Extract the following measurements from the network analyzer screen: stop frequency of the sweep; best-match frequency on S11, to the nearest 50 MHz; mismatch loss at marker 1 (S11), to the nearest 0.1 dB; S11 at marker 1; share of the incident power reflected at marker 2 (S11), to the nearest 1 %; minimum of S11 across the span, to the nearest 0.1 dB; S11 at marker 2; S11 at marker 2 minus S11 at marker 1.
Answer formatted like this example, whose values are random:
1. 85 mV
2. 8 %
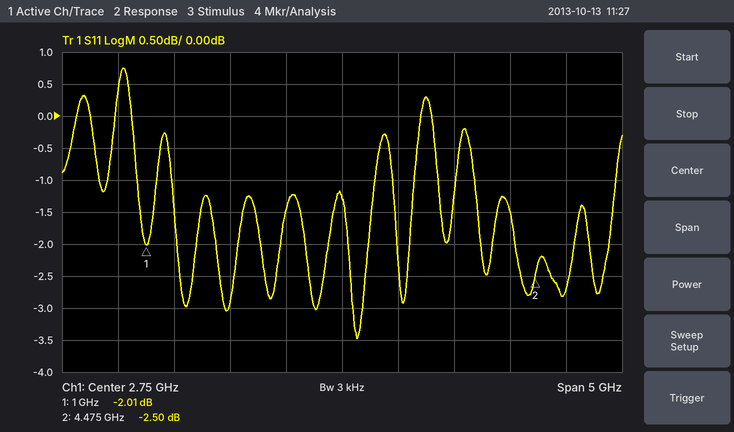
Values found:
1. 5.25 GHz
2. 2.90 GHz
3. 4.3 dB
4. -2.01 dB
5. 56 %
6. -3.5 dB
7. -2.50 dB
8. -0.49 dB
